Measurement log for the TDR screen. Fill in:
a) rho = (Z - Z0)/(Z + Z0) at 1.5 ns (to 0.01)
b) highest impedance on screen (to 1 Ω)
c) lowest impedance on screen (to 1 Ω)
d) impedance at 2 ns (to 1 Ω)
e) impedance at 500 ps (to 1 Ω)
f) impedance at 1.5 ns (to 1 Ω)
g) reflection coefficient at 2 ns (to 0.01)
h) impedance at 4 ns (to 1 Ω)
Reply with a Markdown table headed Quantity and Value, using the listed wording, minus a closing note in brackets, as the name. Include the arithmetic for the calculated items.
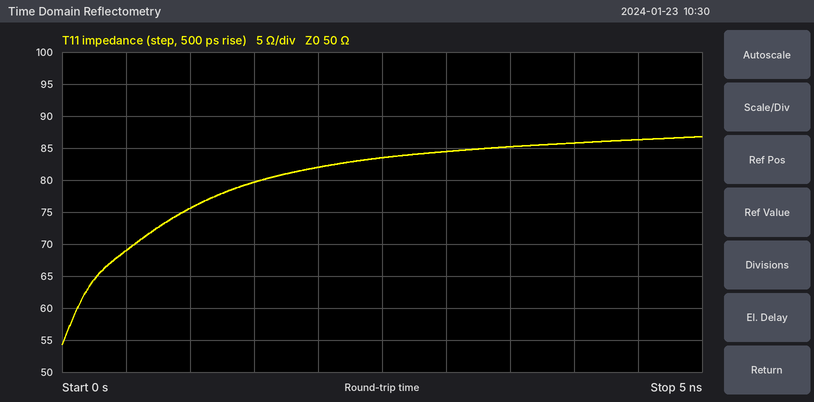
| Quantity | Value |
|---|---|
| rho = (Z - Z0)/(Z + Z0) at 1.5 ns | (80 − 50)/(80 + 50) ≈ +0.23 |
| highest impedance on screen | 87 Ω |
| lowest impedance on screen | 54 Ω |
| impedance at 2 ns | 82 Ω |
| impedance at 500 ps | 69 Ω |
| impedance at 1.5 ns | 80 Ω |
| reflection coefficient at 2 ns | (82 − 50)/(82 + 50) ≈ +0.24 |
| impedance at 4 ns | 86 Ω |
